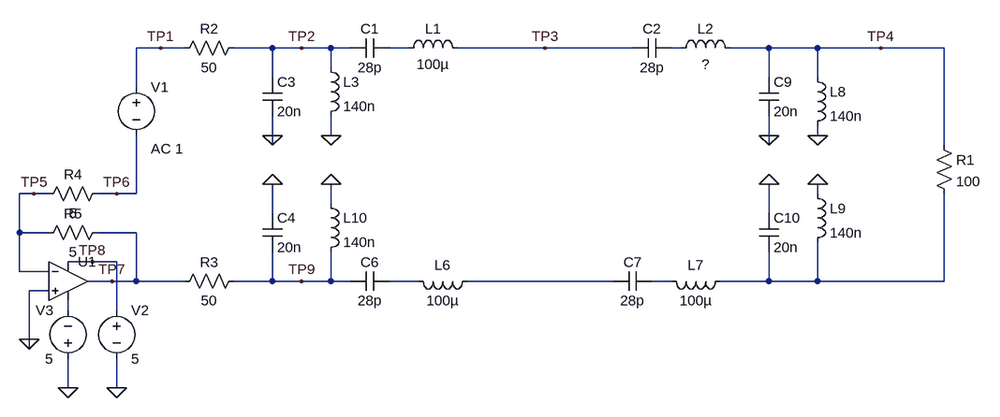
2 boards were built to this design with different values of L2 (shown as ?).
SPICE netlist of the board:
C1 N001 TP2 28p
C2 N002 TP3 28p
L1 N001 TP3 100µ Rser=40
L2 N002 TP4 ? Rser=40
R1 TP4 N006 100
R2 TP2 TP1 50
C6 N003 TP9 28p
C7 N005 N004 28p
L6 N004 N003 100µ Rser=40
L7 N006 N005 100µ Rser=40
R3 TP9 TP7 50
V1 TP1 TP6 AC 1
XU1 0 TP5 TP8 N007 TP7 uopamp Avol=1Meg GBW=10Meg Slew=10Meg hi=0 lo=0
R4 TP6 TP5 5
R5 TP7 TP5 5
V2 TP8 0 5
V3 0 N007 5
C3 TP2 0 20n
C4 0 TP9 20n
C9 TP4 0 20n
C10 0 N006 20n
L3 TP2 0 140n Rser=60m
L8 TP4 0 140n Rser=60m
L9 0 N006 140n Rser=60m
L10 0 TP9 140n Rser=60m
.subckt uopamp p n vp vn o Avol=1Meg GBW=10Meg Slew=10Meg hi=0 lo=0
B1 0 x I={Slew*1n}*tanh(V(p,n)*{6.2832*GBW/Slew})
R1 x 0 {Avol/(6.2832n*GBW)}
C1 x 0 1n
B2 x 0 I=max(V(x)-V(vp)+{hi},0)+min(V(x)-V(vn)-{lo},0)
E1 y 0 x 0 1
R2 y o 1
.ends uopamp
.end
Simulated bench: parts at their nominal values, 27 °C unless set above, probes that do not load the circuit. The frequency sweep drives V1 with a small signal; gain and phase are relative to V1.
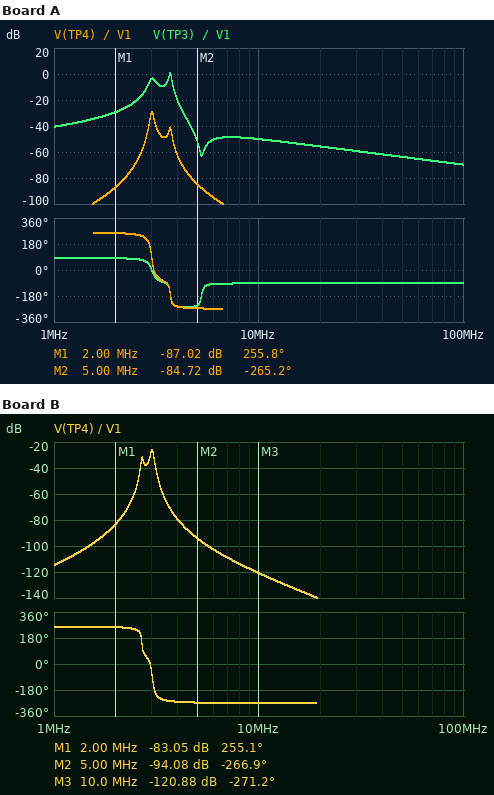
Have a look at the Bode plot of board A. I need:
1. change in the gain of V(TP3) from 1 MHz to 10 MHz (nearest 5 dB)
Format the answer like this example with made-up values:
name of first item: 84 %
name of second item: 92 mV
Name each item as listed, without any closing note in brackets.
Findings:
change in the gain of V(TP3) from 1 MHz to 10 MHz: -10 dB
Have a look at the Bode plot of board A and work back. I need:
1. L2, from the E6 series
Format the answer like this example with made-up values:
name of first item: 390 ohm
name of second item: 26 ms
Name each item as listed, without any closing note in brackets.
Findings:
L2, from the E6 series: 33 µH
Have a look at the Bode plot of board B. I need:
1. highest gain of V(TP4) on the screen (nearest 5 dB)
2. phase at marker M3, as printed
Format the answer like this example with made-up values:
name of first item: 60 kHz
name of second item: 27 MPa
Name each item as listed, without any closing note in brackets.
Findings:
highest gain of V(TP4) on the screen: -25 dB
phase at marker M3, as printed: -271.2 deg
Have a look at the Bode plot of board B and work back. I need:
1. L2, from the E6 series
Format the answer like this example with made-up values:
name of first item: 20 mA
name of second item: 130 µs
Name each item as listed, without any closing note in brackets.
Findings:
L2, from the E6 series: 150 µH
